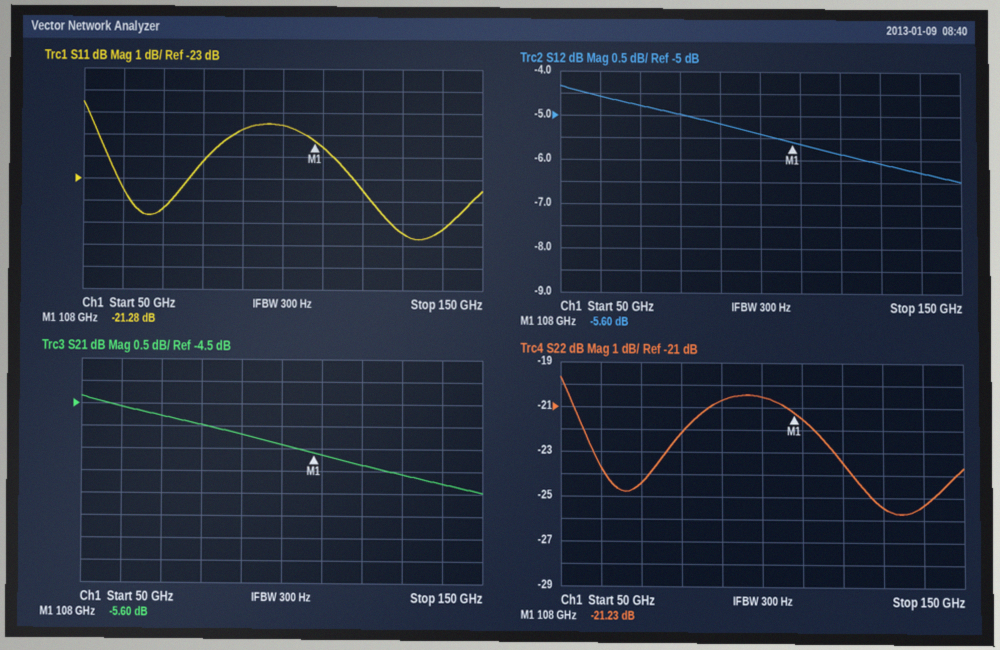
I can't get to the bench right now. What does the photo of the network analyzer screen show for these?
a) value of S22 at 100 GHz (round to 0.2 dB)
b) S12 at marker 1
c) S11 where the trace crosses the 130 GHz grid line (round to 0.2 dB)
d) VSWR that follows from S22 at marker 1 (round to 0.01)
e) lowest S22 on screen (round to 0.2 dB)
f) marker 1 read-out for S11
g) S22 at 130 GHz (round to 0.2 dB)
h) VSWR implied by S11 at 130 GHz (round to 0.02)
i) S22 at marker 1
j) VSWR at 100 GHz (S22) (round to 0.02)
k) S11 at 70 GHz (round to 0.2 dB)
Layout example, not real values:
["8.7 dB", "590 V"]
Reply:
["-20.6 dB", "-5.60 dB", "-25.4 dB", "1.19", "-25.8 dB", "-21.28 dB", "-25.4 dB", "1.12", "-21.23 dB", "1.20", "-24.4 dB"]
